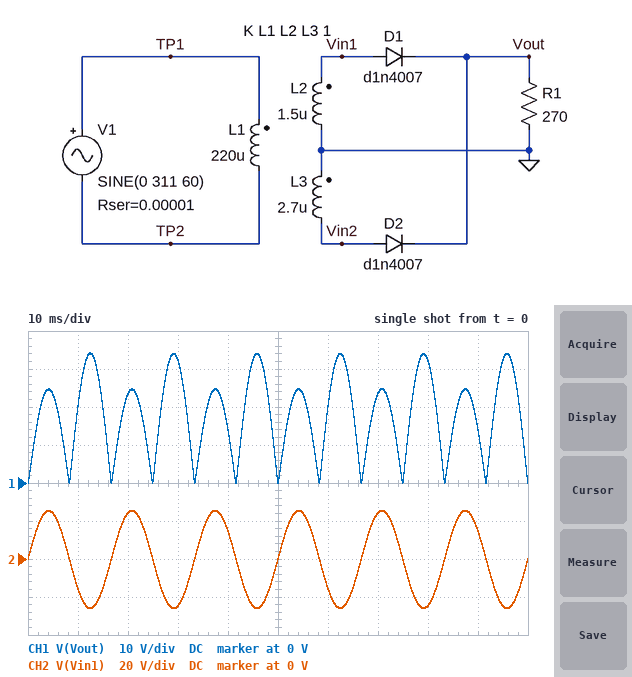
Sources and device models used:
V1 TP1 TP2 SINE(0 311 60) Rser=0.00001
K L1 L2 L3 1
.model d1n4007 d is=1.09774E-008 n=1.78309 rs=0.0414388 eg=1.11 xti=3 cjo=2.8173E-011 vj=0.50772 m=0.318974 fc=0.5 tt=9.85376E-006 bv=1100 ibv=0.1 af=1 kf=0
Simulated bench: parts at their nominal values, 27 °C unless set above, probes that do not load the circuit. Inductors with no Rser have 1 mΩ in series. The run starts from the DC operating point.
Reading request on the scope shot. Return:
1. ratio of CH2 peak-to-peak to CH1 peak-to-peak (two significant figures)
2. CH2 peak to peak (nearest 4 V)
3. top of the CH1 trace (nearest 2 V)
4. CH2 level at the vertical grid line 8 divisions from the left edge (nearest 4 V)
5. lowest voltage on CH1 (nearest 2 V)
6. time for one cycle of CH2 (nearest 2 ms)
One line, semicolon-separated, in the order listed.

1.5; 52 V; 34 V; -24 V; 0 V; 16 ms
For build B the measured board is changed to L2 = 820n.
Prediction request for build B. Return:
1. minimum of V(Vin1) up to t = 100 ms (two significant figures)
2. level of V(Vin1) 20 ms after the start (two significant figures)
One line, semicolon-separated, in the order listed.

-19 V; 18 V
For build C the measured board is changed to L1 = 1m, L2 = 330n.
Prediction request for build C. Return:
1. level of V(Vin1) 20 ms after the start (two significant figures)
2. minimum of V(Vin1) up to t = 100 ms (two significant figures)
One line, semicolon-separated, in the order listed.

5.4 V; -5.7 V
